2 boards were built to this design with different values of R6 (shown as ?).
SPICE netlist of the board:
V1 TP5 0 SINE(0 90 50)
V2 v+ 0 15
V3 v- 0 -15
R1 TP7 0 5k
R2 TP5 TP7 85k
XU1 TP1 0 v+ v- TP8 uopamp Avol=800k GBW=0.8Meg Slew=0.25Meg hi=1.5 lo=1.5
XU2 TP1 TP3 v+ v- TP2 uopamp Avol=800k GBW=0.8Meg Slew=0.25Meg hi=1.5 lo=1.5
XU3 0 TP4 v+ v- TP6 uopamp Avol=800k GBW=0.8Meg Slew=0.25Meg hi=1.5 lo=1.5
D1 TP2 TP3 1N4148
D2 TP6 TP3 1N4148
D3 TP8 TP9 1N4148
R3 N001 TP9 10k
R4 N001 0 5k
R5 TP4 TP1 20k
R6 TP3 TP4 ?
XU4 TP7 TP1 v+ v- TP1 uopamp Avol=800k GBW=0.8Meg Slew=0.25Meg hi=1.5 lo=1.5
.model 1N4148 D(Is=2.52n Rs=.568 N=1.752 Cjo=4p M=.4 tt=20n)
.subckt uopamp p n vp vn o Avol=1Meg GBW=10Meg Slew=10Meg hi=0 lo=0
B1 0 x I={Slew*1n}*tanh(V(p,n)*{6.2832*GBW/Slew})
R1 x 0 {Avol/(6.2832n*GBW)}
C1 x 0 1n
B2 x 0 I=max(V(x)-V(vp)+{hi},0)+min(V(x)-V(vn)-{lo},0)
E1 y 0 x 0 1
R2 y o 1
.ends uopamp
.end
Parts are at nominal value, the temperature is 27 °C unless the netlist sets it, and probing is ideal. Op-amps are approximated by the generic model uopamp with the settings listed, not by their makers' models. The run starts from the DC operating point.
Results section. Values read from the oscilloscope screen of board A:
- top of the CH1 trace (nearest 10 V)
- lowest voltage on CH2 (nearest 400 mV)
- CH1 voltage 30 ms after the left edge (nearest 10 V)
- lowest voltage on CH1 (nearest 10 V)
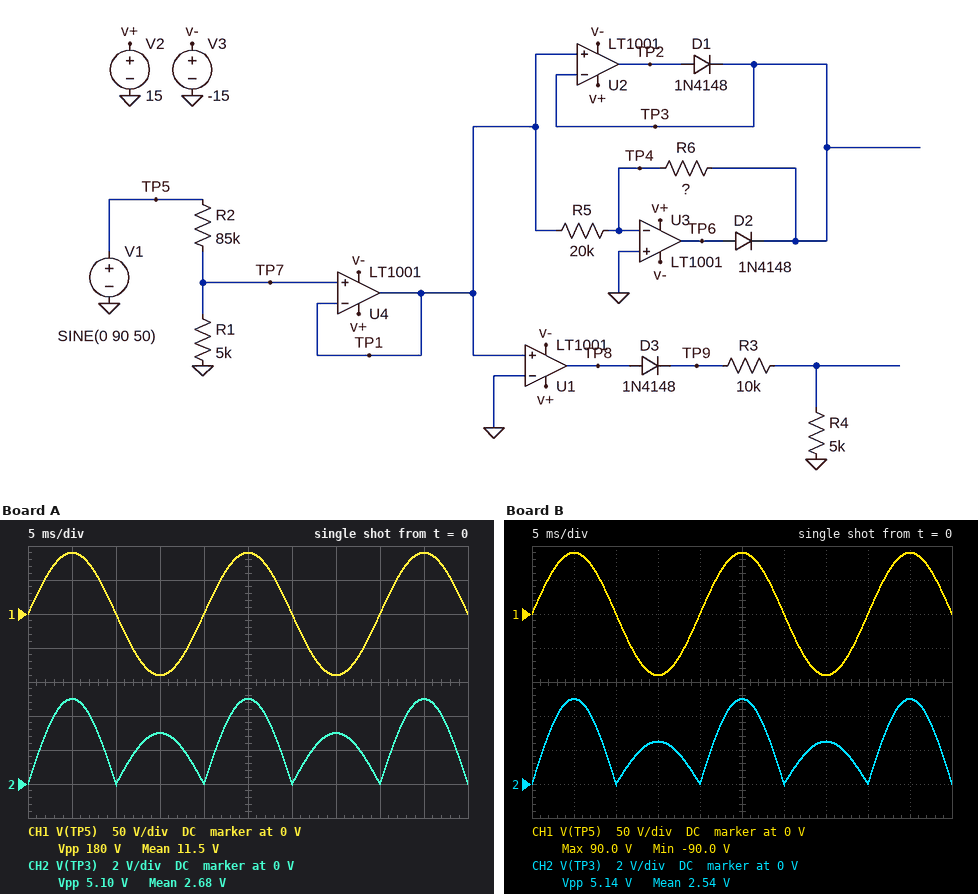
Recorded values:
90 V
0 V
0 V
-90 V
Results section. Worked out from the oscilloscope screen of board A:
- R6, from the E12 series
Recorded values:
12 kΩ
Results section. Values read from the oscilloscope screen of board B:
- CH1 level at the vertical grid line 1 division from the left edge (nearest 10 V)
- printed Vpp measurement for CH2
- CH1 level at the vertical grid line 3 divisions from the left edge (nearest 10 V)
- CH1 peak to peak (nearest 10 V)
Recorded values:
90 V
5.14 V
-90 V
180 V
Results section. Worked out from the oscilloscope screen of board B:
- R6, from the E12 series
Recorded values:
10 kΩ
